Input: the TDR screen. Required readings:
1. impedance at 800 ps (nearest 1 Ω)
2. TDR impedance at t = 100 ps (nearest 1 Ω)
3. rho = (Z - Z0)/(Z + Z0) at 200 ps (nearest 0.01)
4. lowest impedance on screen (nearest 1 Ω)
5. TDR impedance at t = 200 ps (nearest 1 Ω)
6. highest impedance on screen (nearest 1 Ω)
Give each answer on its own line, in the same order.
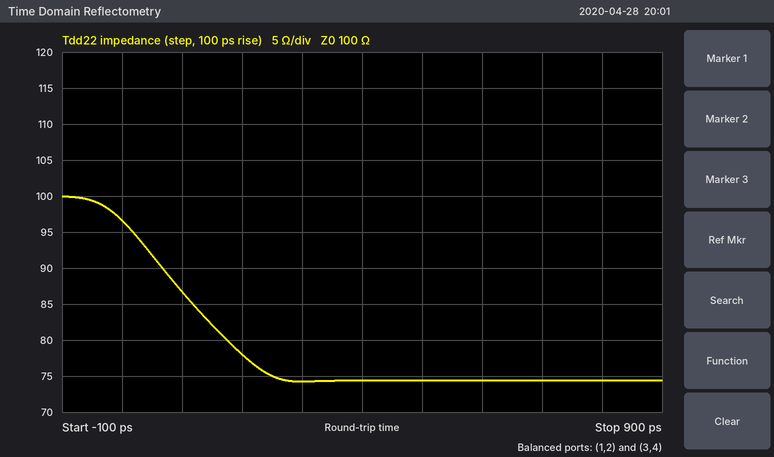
74 Ω
87 Ω
-0.12
74 Ω
78 Ω
100 Ω
